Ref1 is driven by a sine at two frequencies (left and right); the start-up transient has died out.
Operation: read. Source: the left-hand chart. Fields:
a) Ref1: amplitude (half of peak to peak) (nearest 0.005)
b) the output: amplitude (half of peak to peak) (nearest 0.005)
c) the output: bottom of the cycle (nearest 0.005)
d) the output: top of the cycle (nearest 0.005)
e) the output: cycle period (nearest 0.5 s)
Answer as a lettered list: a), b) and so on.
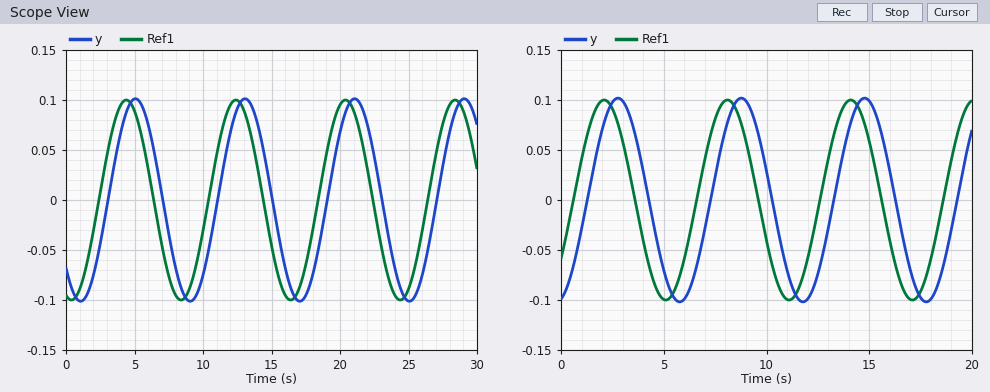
a) 0.100
b) 0.100
c) -0.100
d) 0.100
e) 8.0 s
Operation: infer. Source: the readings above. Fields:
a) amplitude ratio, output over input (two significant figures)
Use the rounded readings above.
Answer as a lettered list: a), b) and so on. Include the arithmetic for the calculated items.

a) 0.1 / 0.1 = 1.0
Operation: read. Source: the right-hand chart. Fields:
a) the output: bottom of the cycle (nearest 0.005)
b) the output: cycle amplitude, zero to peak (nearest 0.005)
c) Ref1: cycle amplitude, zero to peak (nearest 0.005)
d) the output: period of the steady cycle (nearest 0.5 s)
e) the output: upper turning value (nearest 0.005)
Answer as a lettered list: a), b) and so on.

a) -0.100
b) 0.100
c) 0.100
d) 6.0 s
e) 0.100
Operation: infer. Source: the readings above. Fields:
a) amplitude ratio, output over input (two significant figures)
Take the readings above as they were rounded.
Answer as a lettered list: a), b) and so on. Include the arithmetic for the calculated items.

a) 0.1 / 0.1 = 1.0
